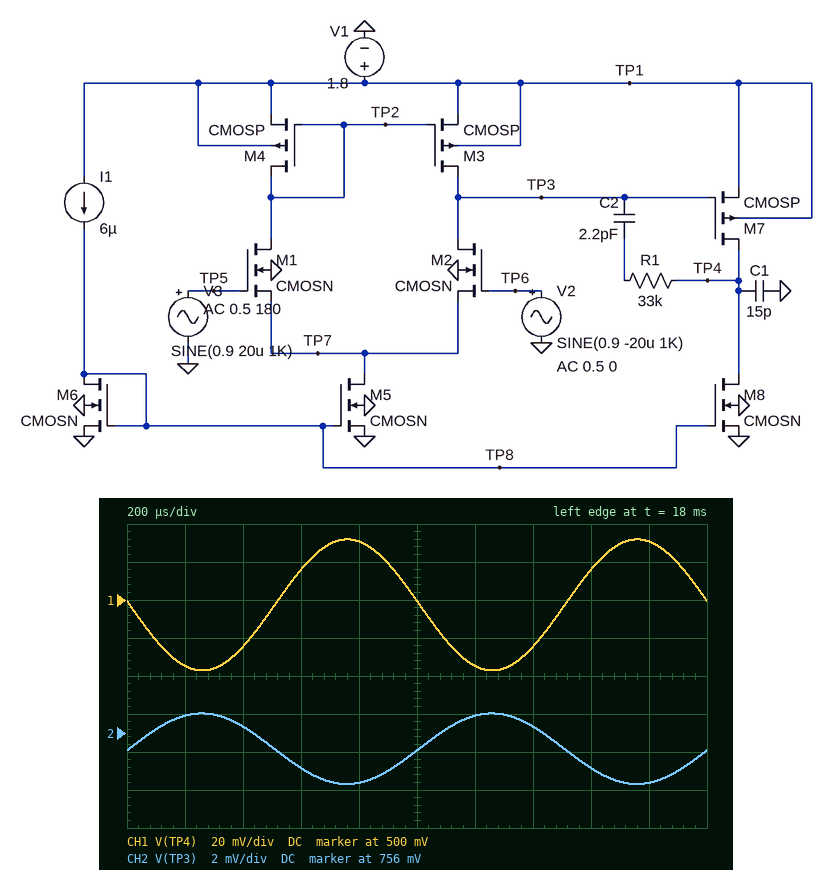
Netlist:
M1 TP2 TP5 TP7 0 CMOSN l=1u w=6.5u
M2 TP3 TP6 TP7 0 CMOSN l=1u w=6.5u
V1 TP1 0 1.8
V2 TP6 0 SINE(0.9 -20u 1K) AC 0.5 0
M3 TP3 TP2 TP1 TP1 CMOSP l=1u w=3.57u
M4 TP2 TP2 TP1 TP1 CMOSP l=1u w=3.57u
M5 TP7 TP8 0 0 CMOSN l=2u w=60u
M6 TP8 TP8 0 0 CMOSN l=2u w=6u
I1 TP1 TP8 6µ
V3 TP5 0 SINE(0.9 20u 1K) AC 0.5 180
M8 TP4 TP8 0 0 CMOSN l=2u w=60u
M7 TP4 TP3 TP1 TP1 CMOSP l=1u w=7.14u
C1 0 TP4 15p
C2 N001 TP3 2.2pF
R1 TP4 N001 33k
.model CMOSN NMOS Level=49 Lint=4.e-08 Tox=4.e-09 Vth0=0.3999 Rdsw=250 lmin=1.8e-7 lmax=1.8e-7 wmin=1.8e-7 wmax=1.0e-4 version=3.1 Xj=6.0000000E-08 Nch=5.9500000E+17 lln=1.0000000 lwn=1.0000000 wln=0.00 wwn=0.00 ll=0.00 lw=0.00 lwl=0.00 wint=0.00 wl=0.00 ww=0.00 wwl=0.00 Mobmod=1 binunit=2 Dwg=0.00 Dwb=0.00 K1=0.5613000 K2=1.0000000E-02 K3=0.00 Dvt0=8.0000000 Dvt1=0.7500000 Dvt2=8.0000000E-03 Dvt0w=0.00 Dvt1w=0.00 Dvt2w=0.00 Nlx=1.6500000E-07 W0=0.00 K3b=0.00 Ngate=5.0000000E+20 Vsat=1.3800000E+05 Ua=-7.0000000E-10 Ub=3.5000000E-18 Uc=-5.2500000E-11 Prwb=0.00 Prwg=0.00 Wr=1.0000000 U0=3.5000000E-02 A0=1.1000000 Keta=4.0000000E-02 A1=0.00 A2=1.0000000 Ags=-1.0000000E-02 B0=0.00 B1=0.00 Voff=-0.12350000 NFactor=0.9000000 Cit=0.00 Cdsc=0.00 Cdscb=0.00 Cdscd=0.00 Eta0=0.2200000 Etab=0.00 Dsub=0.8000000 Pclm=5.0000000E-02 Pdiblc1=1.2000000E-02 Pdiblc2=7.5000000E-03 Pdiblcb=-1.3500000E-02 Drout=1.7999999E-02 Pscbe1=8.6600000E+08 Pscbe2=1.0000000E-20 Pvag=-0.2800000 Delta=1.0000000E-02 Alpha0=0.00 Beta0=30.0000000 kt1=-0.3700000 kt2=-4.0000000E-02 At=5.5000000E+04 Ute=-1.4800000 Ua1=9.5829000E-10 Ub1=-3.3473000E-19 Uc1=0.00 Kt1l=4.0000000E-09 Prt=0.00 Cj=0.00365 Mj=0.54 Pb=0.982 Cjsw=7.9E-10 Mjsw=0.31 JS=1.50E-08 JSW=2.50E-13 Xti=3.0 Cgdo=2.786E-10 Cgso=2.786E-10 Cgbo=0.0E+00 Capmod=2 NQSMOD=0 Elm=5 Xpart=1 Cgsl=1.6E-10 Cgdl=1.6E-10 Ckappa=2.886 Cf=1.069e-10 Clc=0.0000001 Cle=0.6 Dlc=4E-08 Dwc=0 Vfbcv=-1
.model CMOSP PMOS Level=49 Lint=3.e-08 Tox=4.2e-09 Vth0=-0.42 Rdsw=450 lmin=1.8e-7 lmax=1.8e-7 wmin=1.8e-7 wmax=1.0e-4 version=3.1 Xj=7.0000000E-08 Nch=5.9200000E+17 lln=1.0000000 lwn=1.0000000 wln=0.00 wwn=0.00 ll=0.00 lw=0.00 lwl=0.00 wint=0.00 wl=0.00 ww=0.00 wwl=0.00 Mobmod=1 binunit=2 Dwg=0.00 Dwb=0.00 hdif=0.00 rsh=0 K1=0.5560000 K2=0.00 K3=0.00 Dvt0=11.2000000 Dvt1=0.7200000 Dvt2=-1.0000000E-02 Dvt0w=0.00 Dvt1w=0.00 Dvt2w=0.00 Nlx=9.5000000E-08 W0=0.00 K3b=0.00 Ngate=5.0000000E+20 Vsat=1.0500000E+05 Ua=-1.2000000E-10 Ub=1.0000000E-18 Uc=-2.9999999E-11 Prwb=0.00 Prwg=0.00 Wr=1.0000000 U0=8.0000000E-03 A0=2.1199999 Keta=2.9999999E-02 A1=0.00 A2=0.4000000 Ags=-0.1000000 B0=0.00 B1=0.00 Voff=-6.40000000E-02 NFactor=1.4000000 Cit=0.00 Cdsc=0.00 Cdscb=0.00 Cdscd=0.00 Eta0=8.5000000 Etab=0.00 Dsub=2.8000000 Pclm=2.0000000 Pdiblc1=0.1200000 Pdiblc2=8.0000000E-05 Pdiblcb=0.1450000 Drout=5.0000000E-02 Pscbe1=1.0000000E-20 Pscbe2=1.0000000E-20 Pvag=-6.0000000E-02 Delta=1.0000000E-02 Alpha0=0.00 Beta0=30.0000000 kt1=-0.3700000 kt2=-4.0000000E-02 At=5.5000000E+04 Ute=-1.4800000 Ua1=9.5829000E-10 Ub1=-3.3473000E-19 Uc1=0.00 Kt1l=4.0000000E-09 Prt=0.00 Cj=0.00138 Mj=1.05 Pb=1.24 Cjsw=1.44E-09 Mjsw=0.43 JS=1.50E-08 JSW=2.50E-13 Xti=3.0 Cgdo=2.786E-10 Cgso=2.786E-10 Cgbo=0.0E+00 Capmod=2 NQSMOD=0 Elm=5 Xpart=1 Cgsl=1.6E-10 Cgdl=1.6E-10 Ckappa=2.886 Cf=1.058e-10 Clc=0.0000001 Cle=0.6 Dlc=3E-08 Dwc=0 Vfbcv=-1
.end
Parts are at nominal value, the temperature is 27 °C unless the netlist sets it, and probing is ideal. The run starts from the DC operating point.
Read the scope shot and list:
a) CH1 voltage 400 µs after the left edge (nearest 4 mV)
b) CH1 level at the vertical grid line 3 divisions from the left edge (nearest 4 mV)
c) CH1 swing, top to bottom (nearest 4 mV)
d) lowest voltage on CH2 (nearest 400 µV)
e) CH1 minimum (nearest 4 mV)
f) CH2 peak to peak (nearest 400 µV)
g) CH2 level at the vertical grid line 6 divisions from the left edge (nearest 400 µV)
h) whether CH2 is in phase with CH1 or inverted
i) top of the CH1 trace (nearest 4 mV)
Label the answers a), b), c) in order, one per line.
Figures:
a) 476 mV
b) 516 mV
c) 68 mV
d) 753.2 mV
e) 464 mV
f) 3.6 mV
g) 756.8 mV
h) inverted
i) 532 mV
